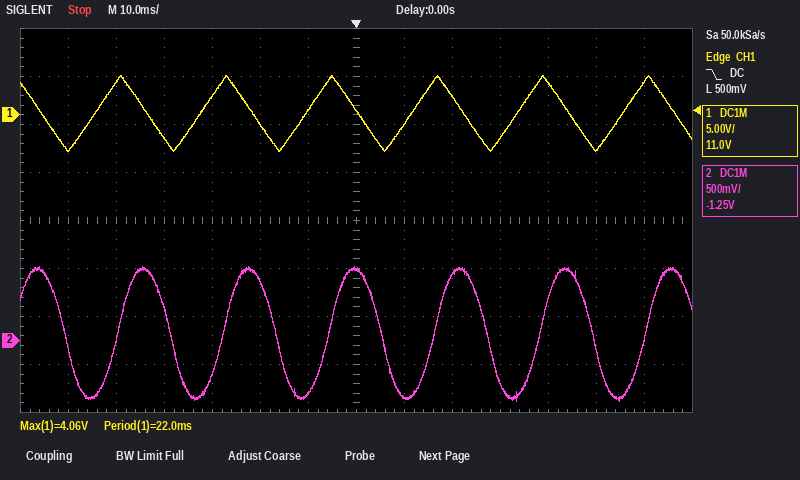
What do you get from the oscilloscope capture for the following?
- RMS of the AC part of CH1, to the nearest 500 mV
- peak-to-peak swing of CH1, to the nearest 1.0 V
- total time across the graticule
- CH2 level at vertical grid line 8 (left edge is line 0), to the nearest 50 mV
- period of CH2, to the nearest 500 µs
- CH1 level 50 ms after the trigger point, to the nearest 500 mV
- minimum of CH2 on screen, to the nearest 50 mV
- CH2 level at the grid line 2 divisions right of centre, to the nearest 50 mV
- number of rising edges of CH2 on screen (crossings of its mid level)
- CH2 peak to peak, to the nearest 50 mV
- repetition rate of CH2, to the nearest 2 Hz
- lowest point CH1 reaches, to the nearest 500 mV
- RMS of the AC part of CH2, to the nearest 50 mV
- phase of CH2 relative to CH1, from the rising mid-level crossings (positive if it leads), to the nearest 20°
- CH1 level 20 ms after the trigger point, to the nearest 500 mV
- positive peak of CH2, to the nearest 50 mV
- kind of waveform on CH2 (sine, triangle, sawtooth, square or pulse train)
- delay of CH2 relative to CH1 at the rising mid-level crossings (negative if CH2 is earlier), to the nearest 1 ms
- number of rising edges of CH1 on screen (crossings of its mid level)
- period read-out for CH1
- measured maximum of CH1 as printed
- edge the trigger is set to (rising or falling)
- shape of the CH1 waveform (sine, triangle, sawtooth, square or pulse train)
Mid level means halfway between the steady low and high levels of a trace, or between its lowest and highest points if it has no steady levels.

2.5 V
8.0 V
140 ms
-600 mV
22.0 ms
-3.5 V
-650 mV
700 mV
6
1.40 V
46 Hz
-4.0 V
500 mV
-80°
2.0 V
750 mV
sine
+5 ms
6
22.0 ms
4.06 V
falling
triangle
